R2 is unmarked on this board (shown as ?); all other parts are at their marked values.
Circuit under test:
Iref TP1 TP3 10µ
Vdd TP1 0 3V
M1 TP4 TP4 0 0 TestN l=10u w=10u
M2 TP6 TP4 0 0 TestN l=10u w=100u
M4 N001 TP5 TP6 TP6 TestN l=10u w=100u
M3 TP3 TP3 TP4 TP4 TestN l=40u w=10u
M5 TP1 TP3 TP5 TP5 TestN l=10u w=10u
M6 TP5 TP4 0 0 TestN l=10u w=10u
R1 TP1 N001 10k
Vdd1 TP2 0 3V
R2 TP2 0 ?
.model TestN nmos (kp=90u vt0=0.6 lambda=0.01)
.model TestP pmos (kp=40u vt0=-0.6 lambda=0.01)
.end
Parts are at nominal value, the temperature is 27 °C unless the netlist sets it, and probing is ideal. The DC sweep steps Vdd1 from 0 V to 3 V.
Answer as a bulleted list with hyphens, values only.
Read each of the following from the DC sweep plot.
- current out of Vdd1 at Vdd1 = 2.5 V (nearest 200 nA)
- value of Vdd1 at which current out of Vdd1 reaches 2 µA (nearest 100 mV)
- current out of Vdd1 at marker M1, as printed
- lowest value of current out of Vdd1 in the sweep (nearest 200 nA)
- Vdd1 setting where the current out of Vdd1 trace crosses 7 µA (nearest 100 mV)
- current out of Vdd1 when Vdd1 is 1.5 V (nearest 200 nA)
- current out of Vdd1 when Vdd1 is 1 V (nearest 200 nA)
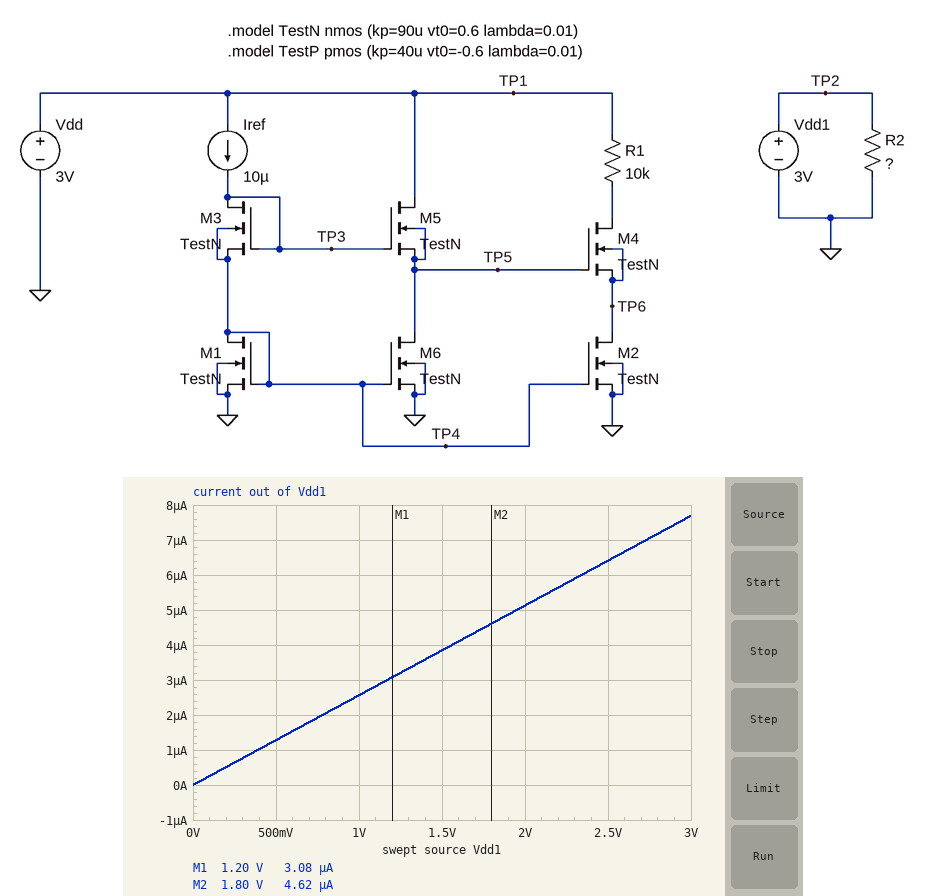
- 6.4 µA
- 800 mV
- 3.08 µA
- 0 A
- 2.7 V
- 3.8 µA
- 2.6 µA
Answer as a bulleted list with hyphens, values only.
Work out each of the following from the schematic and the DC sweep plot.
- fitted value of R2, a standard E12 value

- 390 kΩ
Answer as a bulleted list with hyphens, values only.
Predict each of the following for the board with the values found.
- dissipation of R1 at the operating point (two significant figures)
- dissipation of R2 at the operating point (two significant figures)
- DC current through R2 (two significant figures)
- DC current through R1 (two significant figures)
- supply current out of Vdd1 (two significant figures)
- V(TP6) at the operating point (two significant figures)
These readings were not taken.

- 99 µW
- 23 µW
- 7.7 µA
- 99 µA
- 7.7 µA
- 470 mV
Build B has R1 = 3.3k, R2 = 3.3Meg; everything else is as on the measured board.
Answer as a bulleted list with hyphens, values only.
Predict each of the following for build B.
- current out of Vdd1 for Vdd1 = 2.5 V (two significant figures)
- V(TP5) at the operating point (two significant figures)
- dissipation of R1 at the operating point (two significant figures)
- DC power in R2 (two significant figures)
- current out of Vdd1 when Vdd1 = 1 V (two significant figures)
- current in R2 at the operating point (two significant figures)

- 760 nA
- 1.5 V
- 33 µW
- 2.7 µW
- 300 nA
- 910 nA
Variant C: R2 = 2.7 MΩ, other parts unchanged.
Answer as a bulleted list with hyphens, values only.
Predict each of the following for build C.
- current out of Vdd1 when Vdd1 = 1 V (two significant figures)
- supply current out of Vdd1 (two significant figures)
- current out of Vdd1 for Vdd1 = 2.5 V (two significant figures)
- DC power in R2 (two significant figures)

- 370 nA
- 1.1 µA
- 930 nA
- 3.3 µW
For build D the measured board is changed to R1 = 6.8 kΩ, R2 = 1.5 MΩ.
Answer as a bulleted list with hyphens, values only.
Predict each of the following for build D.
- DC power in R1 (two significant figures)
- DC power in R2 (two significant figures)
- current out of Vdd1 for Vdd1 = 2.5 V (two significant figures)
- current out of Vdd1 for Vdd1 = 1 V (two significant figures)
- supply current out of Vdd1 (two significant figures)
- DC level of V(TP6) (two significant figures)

- 67 µW
- 6.0 µW
- 1.7 µA
- 670 nA
- 2.0 µA
- 470 mV
